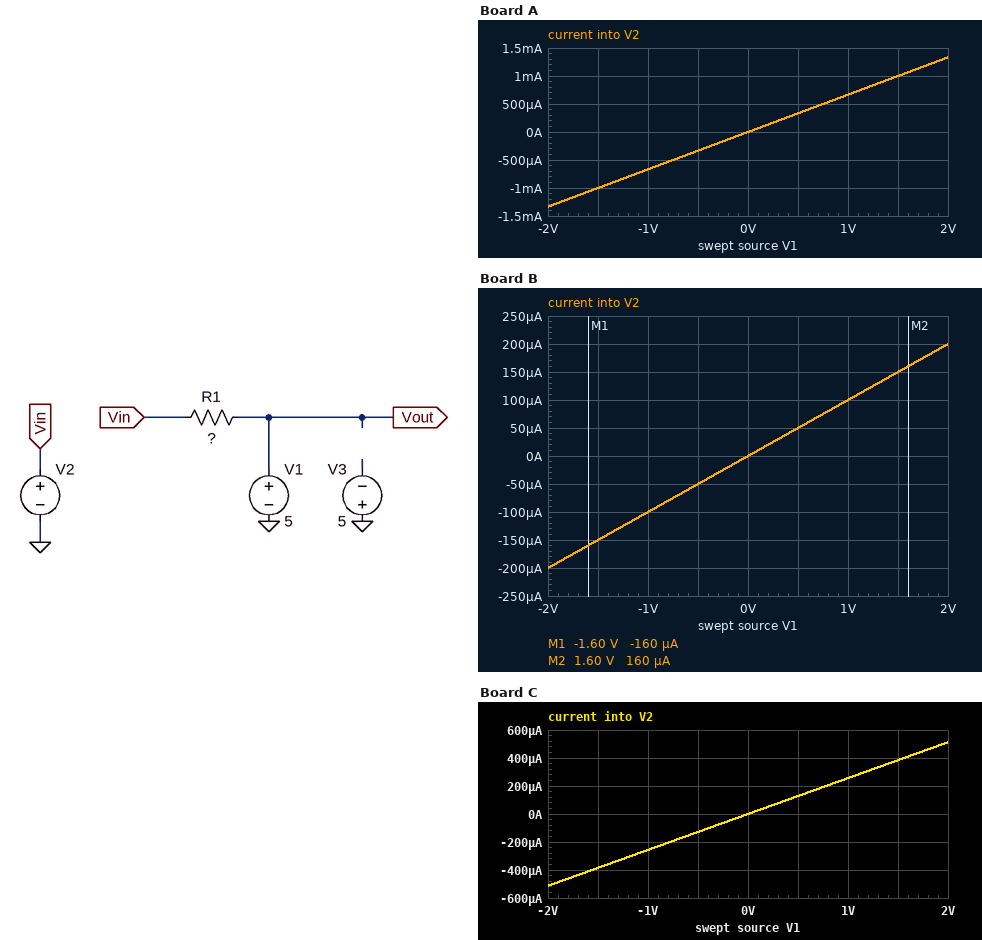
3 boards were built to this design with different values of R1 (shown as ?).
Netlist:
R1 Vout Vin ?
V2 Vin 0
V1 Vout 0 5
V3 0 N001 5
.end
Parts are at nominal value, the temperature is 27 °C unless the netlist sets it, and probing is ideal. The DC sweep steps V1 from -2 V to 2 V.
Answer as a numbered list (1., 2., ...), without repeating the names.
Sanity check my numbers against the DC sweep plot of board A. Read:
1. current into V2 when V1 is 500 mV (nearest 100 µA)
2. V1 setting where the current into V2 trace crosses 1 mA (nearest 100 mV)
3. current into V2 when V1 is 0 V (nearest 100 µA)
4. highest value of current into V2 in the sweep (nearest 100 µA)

1. 300 µA
2. 1.5 V
3. 0 A
4. 1.3 mA
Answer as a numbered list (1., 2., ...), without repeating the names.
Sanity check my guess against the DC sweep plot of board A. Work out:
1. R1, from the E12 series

1. 1.5 kΩ
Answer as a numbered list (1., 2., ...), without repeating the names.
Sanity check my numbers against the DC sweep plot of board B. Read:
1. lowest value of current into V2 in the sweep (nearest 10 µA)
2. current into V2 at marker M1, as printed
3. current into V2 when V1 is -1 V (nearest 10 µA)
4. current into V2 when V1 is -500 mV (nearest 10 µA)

1. -200 µA
2. -160 µA
3. -100 µA
4. -50 µA
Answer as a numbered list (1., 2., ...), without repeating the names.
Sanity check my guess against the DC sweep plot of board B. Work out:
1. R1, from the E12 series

1. 10 kΩ
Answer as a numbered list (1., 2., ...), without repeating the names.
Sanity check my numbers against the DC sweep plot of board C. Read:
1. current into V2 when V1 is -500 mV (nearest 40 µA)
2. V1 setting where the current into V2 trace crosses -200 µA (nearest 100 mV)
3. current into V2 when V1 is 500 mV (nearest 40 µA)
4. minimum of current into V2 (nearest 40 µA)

1. -120 µA
2. -800 mV
3. 120 µA
4. -520 µA
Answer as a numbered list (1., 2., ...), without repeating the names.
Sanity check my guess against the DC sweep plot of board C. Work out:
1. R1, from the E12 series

1. 3.9 kΩ
